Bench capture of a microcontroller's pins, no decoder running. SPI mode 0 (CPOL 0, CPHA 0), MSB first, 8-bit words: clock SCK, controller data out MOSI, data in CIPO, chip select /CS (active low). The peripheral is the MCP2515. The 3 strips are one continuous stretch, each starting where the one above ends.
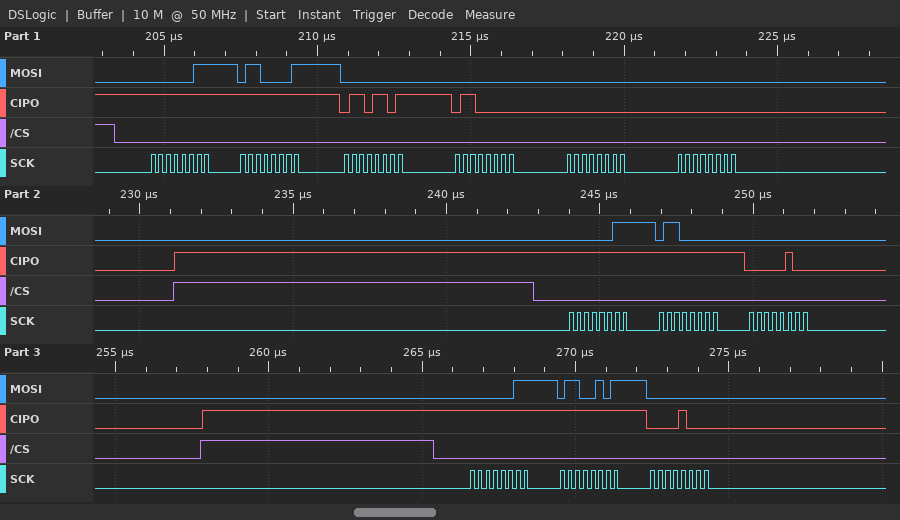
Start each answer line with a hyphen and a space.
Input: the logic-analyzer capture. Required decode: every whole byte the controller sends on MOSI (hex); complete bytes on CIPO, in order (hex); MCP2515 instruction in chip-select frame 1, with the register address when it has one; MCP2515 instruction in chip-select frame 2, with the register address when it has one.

- 03 61 00 00 00 00 03 60 00 03 65 00
- FF FF 6D 60 00 00 FF FF 04 FF FF 08
- READ 0x61
- READ 0x60
